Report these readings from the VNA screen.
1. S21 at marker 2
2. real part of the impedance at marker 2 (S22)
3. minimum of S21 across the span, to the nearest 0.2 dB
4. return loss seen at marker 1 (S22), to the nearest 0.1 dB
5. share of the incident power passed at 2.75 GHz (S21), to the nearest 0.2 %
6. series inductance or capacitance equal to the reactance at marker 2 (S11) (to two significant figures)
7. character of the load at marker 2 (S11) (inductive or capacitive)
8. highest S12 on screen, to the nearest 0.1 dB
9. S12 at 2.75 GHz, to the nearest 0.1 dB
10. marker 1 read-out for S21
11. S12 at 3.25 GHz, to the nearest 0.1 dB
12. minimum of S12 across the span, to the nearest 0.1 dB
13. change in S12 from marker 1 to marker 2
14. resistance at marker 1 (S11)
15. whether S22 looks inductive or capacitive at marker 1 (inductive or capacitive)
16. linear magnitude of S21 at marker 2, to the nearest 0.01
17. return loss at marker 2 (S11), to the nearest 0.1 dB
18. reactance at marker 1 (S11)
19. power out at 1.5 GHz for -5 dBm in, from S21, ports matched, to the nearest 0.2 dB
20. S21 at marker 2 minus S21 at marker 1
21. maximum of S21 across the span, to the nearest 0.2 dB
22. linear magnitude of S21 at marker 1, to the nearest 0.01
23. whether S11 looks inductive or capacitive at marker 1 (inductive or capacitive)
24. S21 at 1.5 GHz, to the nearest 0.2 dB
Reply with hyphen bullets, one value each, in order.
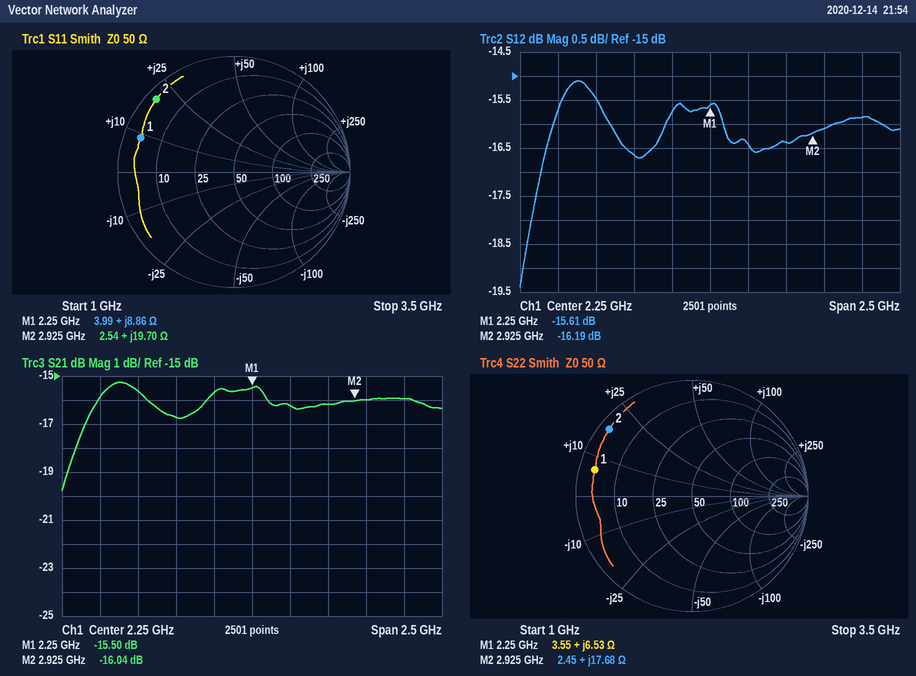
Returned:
- -16.04 dB
- 2.45 Ω
- -19.8 dB
- 1.2 dB
- 2.4 %
- 1.1 nH
- inductive
- -15.1 dB
- -16.4 dB
- -15.50 dB
- -15.9 dB
- -19.4 dB
- -0.58 dB
- 3.99 Ω
- inductive
- 0.16
- 0.8 dB
- +8.86 Ω
- -20.6 dBm
- -0.54 dB
- -15.2 dB
- 0.17
- inductive
- -15.6 dB
